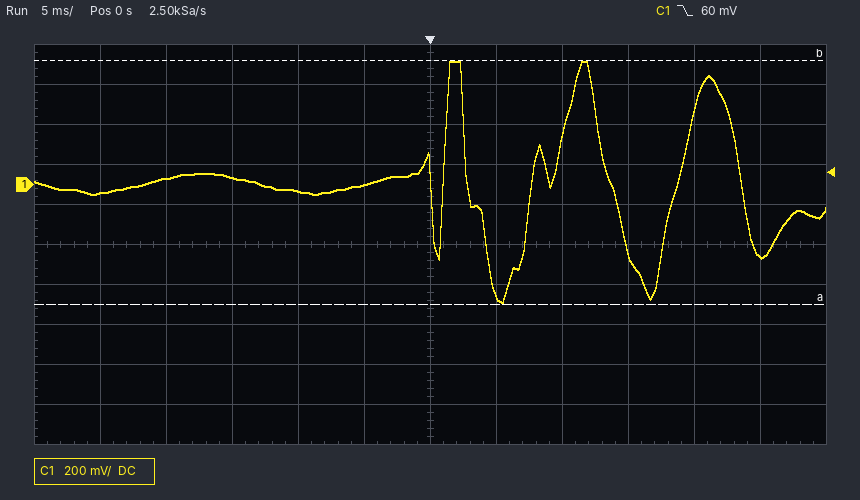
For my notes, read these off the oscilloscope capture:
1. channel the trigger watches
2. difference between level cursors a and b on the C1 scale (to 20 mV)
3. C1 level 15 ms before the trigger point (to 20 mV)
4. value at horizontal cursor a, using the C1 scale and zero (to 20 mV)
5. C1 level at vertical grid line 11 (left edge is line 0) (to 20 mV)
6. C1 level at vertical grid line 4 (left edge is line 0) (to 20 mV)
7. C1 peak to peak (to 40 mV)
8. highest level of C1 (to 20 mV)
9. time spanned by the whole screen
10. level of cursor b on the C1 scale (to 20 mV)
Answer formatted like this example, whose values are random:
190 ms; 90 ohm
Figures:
C1; 1.22 V; 40 mV; -600 mV; -360 mV; -40 mV; 1.20 V; 620 mV; 60 ms; 620 mV
